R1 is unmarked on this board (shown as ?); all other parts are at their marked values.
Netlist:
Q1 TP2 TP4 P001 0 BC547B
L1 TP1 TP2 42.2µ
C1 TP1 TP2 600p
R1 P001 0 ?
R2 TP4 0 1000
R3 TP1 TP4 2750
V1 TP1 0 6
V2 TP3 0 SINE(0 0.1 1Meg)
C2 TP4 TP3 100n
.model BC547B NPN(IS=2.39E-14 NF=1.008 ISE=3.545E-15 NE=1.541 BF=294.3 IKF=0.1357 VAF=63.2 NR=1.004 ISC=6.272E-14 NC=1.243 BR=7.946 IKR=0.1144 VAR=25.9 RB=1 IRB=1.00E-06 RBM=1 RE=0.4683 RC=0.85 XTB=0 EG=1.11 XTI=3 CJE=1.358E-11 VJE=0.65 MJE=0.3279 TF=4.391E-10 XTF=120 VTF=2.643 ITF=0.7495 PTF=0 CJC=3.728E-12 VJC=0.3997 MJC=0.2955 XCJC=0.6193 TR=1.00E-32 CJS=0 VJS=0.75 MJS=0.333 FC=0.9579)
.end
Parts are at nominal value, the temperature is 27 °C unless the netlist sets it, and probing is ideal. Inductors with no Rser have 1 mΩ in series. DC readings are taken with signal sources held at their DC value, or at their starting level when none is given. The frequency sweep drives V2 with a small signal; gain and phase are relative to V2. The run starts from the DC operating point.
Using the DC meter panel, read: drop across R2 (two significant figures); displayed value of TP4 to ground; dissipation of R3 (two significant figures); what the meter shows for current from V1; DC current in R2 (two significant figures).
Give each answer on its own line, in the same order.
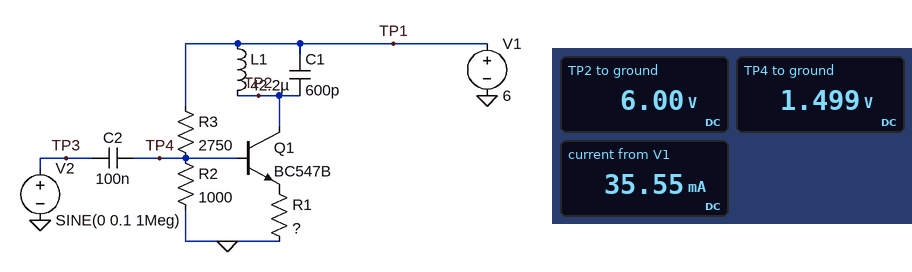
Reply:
1.5 V
1.499 V
7.4 mW
35.55 mA
1.5 mA
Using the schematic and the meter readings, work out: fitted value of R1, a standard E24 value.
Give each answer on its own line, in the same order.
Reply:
22 Ω
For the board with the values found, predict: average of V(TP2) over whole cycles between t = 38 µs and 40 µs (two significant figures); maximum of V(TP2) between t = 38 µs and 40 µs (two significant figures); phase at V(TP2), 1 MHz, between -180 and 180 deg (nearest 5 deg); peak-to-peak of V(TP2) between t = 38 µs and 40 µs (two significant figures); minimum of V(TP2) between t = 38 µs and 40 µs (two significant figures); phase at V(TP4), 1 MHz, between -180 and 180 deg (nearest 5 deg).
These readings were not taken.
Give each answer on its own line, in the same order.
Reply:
6.0 V
13 V
150 deg
13 V
330 mV
0 deg
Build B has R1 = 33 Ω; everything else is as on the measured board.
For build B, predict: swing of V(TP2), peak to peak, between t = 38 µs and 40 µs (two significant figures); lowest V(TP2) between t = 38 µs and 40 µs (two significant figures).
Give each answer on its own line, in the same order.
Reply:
12 V
520 mV
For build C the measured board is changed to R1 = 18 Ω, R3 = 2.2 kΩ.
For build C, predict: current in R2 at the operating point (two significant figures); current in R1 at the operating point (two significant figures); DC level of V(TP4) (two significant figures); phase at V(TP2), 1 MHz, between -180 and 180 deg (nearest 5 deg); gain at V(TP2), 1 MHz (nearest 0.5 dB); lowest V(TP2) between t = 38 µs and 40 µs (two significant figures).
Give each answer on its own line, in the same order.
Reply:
1.7 mA
52 mA
1.7 V
145 deg
62.5 dB
440 mV
